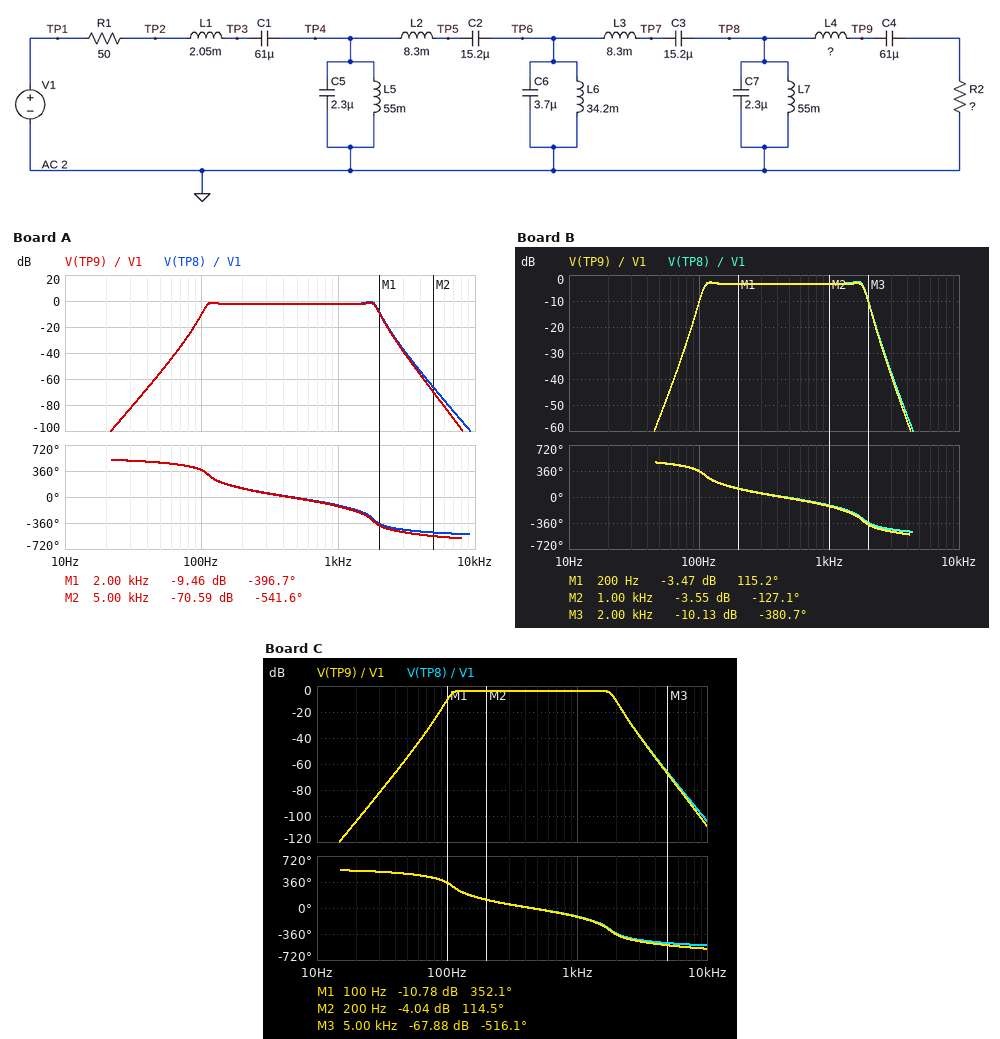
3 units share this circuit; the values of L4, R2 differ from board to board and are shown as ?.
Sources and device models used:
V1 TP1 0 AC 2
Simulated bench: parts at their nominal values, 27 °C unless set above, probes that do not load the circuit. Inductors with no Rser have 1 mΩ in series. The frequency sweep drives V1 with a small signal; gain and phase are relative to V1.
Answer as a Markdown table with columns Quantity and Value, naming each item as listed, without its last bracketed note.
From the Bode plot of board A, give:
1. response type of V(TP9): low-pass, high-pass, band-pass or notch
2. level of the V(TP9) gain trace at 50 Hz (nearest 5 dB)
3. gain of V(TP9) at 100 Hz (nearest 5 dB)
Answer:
| Quantity | Value |
|---|---|
| response type of V(TP9): low-pass, high-pass, band-pass or notch | band-pass |
| level of the V(TP9) gain trace at 50 Hz | -55 dB |
| gain of V(TP9) at 100 Hz | -10 dB |
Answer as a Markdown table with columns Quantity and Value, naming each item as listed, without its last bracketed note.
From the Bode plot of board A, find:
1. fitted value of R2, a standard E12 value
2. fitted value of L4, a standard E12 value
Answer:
| Quantity | Value |
|---|---|
| fitted value of R2, a standard E12 value | 150 Ω |
| fitted value of L4, a standard E12 value | 5.6 mH |
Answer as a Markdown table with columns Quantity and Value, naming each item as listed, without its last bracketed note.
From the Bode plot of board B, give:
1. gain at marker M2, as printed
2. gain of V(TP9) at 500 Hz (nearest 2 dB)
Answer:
| Quantity | Value |
|---|---|
| gain at marker M2, as printed | -3.55 dB |
| gain of V(TP9) at 500 Hz | -4 dB |
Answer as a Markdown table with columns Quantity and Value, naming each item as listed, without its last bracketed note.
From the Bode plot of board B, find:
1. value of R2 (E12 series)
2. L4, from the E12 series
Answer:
| Quantity | Value |
|---|---|
| value of R2 | 100 Ω |
| L4, from the E12 series | 3.3 mH |
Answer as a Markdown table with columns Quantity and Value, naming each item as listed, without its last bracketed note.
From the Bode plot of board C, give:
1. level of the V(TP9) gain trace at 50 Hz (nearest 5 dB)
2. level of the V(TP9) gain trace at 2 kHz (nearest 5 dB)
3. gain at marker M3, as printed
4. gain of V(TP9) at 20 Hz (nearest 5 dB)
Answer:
| Quantity | Value |
|---|---|
| level of the V(TP9) gain trace at 50 Hz | -55 dB |
| level of the V(TP9) gain trace at 2 kHz | -10 dB |
| gain at marker M3, as printed | -67.88 dB |
| gain of V(TP9) at 20 Hz | -105 dB |
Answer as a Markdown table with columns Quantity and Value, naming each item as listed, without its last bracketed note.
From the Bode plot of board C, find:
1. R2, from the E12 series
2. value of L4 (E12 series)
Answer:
| Quantity | Value |
|---|---|
| R2, from the E12 series | 82 Ω |
| value of L4 | 1.5 mH |
